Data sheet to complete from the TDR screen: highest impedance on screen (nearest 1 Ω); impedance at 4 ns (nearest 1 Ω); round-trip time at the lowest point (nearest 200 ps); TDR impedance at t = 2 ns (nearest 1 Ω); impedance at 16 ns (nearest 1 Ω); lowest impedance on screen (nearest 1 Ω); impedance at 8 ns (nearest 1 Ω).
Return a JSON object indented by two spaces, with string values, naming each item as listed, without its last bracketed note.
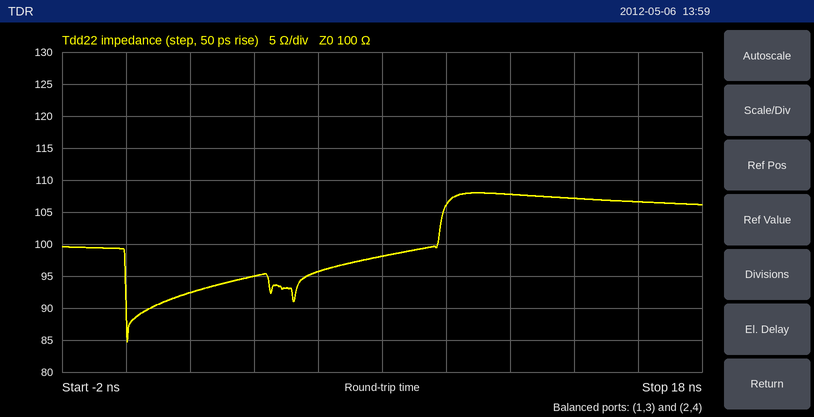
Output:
{
  "highest impedance on screen": "108 Ω",
  "impedance at 4 ns": "95 Ω",
  "round-trip time at the lowest point": "0.0 ns",
  "TDR impedance at t = 2 ns": "92 Ω",
  "impedance at 16 ns": "107 Ω",
  "lowest impedance on screen": "85 Ω",
  "impedance at 8 ns": "98 Ω"
}
